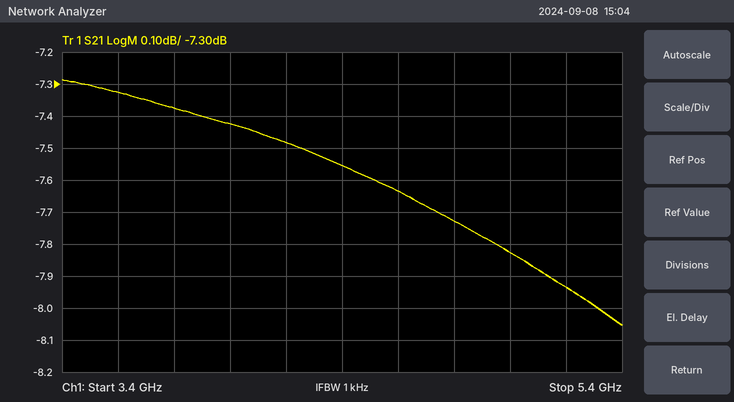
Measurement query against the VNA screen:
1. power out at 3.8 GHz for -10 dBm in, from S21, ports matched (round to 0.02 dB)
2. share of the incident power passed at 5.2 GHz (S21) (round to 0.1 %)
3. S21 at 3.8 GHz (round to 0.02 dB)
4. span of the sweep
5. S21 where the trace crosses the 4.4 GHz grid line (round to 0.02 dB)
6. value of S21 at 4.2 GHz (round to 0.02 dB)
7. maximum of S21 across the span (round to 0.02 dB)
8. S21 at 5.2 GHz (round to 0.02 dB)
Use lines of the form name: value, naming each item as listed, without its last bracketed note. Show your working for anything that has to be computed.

power out at 3.8 GHz for -10 dBm in, from S21, ports matched: -10 dBm + (-7.38 dB) = -17.38 dBm
share of the incident power passed at 5.2 GHz (S21): 10^(-7.94/10) ≈ 16.1 %
S21 at 3.8 GHz: -7.38 dB
span of the sweep: 2 GHz
S21 where the trace crosses the 4.4 GHz grid line: -7.56 dB
value of S21 at 4.2 GHz: -7.48 dB
maximum of S21 across the span: -7.28 dB
S21 at 5.2 GHz: -7.94 dB
